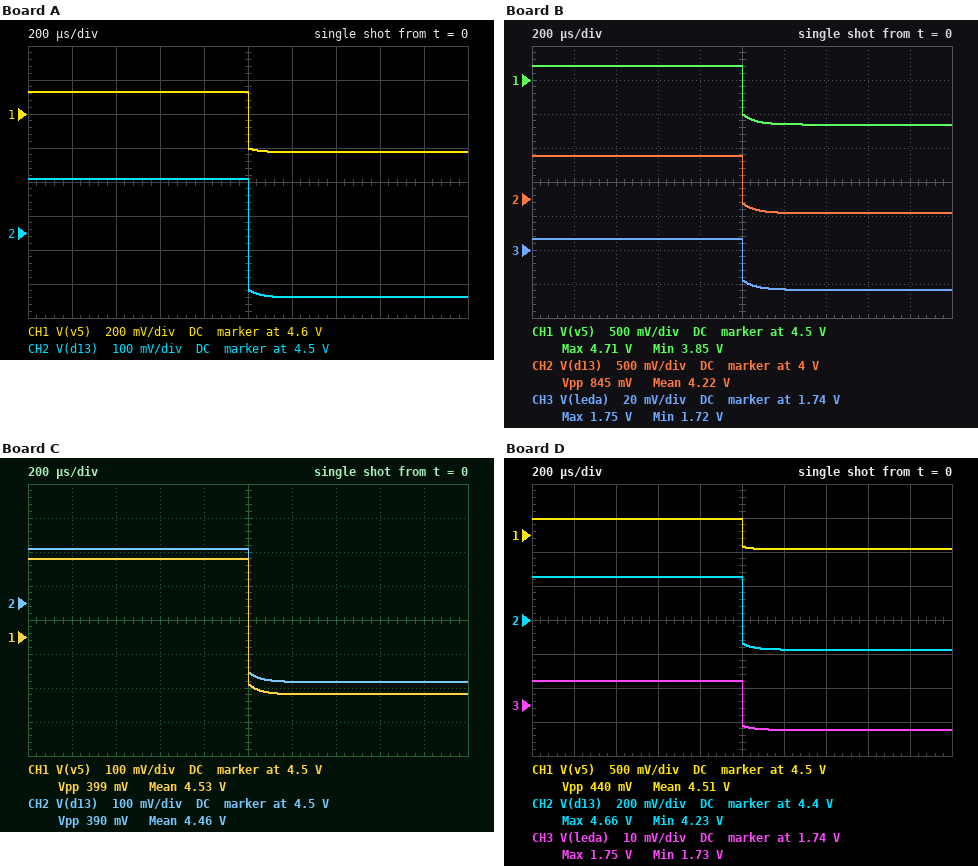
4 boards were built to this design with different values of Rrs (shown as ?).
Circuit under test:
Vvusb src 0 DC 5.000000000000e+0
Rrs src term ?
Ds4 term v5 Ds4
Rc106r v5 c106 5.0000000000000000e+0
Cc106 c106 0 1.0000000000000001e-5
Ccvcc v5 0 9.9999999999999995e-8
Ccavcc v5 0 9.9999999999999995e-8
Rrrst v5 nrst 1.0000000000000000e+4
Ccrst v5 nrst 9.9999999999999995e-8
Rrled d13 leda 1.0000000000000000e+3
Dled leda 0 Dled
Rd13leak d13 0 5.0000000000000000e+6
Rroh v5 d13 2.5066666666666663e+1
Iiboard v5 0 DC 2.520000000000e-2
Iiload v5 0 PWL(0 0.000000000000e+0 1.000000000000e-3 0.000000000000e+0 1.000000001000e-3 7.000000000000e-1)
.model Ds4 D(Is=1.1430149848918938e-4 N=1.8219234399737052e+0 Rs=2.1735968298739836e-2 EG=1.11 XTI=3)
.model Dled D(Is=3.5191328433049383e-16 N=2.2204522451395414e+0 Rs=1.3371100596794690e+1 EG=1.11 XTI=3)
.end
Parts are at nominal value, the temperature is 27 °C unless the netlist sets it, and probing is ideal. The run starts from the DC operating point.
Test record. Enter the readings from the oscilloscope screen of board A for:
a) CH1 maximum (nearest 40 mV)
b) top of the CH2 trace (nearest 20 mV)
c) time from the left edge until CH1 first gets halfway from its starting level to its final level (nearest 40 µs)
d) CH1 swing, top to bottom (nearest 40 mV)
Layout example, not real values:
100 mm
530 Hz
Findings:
4.72 V
4.66 V
1.00 ms
360 mV
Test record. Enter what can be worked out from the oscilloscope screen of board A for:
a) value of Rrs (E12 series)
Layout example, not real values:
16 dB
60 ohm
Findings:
0.27 Ω
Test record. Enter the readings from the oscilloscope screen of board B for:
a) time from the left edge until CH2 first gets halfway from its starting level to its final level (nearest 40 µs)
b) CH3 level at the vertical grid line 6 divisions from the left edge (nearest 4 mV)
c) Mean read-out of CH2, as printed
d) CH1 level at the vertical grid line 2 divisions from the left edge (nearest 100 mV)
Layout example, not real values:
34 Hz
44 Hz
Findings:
1.00 ms
1.716 V
4.22 V
4.7 V
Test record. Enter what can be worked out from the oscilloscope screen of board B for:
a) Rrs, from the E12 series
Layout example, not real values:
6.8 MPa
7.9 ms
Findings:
1 Ω
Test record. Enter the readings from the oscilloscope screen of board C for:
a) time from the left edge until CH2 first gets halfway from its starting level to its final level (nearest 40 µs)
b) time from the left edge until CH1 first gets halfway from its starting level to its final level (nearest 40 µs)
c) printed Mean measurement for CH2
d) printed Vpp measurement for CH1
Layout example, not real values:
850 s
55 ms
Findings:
1.00 ms
1.00 ms
4.46 V
399 mV
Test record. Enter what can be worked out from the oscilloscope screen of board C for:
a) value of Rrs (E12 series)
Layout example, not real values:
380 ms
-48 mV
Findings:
0.33 Ω
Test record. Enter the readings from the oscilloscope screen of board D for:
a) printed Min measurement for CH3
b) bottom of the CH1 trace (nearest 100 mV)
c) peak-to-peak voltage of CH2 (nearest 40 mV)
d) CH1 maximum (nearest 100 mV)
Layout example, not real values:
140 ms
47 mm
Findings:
1.73 V
4.3 V
440 mV
4.7 V
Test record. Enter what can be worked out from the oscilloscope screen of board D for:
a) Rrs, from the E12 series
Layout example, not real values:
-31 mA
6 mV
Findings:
0.39 Ω
